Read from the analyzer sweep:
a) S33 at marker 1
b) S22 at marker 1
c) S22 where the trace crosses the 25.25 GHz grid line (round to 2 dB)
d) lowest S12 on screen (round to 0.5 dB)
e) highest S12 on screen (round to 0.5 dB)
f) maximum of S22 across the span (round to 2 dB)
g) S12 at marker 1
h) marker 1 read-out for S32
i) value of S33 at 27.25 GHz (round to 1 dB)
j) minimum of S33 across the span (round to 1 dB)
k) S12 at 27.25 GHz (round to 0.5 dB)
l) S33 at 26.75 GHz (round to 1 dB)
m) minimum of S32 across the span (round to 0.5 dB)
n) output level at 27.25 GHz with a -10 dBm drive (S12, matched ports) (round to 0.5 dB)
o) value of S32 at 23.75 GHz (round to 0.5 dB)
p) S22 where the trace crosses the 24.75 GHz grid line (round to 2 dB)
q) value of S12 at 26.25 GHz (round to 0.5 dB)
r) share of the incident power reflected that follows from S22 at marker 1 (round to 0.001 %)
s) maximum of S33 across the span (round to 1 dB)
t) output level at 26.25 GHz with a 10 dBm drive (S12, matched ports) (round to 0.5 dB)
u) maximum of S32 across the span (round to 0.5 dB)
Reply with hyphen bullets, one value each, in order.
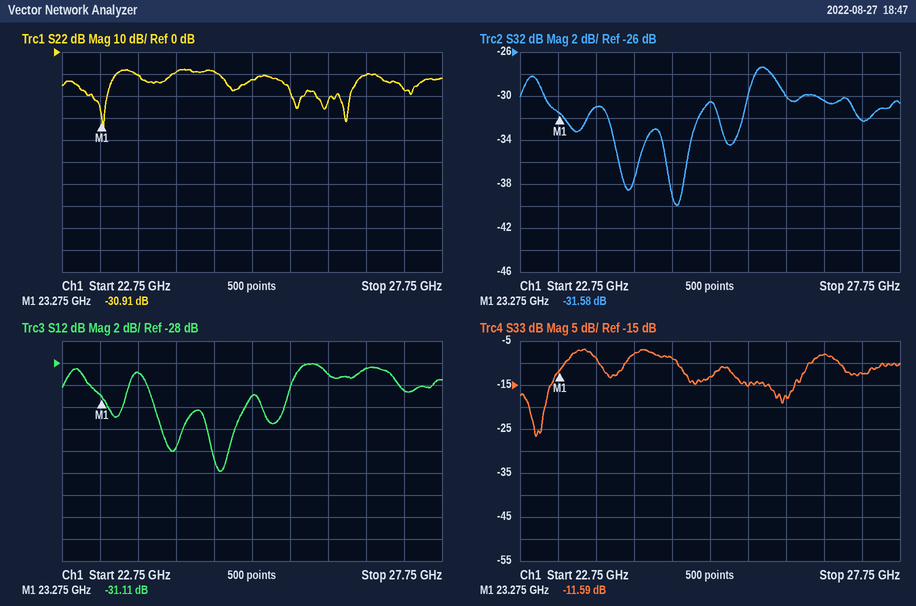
- -11.59 dB
- -30.91 dB
- -12 dB
- -38.0 dB
- -28.0 dB
- -8 dB
- -31.11 dB
- -31.58 dB
- -12 dB
- -27 dB
- -30.5 dB
- -8 dB
- -40.0 dB
- -40.5 dBm
- -31.0 dB
- -8 dB
- -29.0 dB
- 0.081 %
- -7 dB
- -19.0 dBm
- -27.5 dB
